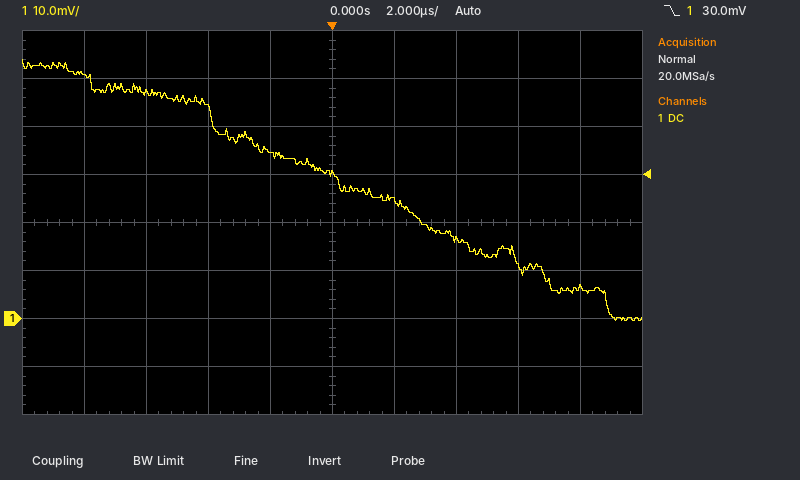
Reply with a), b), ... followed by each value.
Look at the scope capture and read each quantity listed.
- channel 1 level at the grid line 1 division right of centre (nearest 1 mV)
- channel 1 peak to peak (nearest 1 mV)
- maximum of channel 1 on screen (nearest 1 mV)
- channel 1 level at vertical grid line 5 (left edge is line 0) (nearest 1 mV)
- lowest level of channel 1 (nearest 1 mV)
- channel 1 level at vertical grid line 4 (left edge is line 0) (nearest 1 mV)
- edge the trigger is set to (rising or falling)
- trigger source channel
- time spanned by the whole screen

a) 25 mV
b) 54 mV
c) 54 mV
d) 30 mV
e) 0 mV
f) 35 mV
g) falling
h) channel 1
i) 20 µs
